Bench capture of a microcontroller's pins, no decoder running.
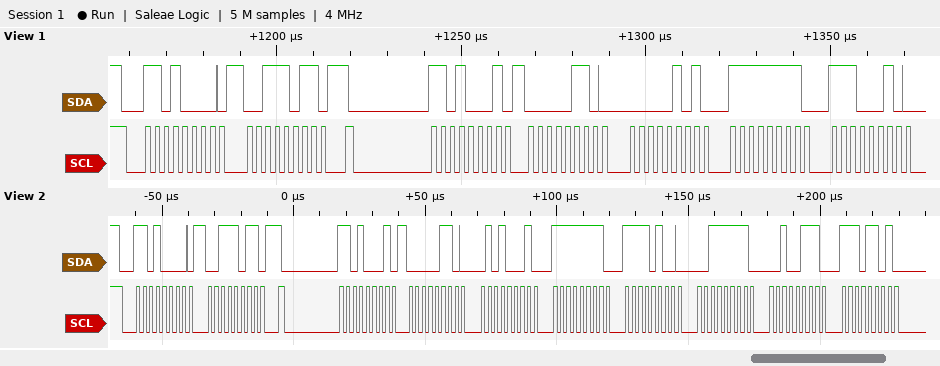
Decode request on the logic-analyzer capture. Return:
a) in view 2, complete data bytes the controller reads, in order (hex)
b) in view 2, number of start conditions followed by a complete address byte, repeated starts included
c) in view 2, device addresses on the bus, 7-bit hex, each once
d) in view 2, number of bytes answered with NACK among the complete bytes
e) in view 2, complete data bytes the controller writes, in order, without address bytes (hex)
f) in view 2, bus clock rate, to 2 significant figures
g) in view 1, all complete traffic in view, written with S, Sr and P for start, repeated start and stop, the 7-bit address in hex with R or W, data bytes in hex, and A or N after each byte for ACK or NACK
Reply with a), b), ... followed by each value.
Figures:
a) 06 51 FF F4 3F 27 ED
b) 2
c) 0x68
d) 0
e) 3B
f) 400 kHz
g) S 68W A 3B A Sr 68R A 06 A 05 A FF A E2 A
